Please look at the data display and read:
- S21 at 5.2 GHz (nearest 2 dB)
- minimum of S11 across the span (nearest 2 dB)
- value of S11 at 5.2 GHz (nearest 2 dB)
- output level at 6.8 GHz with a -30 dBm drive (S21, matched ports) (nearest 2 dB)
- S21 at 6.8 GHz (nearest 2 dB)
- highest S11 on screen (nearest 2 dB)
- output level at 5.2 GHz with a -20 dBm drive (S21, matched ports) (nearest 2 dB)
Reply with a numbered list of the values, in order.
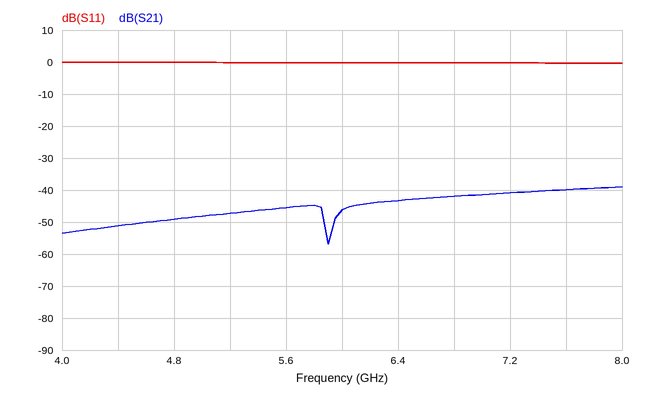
1. -48 dB
2. 0 dB
3. 0 dB
4. -72 dBm
5. -42 dB
6. 0 dB
7. -68 dBm
